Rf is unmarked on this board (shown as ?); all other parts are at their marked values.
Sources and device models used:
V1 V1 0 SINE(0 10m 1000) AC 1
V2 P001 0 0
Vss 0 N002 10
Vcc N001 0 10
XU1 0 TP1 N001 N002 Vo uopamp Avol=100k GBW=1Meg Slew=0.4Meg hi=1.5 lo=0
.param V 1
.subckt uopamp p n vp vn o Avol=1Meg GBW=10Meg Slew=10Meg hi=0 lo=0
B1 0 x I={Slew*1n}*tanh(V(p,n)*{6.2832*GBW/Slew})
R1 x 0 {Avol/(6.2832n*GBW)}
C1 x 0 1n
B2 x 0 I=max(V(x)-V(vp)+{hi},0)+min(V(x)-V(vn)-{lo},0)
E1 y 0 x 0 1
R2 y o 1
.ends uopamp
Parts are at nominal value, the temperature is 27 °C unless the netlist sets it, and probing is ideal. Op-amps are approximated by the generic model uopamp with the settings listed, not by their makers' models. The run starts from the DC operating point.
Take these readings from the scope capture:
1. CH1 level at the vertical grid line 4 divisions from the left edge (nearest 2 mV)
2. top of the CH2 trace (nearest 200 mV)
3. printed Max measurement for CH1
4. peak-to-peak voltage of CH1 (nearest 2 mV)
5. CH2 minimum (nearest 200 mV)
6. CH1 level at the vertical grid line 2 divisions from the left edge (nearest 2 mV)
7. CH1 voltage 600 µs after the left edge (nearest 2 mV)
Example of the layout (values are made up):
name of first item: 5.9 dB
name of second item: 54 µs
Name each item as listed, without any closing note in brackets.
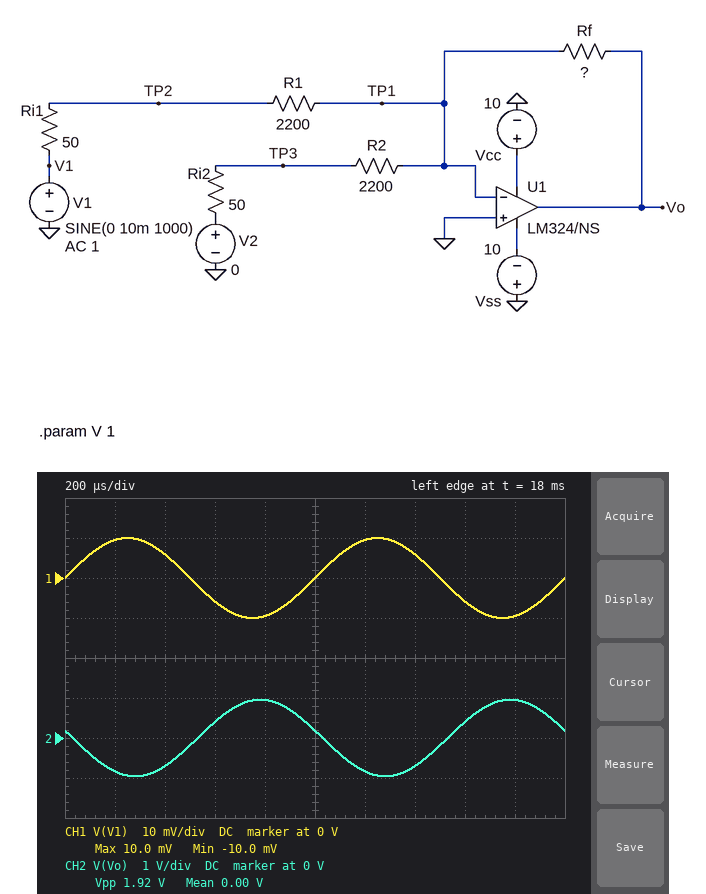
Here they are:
CH1 level at the vertical grid line 4 divisions from the left edge: -10 mV
top of the CH2 trace: 1.0 V
printed Max measurement for CH1: 10.0 mV
peak-to-peak voltage of CH1: 20 mV
CH2 minimum: -1.0 V
CH1 level at the vertical grid line 2 divisions from the left edge: 6 mV
CH1 voltage 600 µs after the left edge: -6 mV
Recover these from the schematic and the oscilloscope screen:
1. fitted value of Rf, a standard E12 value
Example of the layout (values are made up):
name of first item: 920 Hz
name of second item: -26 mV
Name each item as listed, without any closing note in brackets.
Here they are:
fitted value of Rf, a standard E12 value: 220 kΩ
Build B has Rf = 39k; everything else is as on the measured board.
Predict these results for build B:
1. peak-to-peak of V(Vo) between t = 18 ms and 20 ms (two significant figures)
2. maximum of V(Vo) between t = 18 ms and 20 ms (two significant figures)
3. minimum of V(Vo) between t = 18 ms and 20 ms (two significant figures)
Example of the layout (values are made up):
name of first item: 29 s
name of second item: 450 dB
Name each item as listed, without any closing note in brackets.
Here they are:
peak-to-peak of V(Vo) between t = 18 ms and 20 ms: 350 mV
maximum of V(Vo) between t = 18 ms and 20 ms: 170 mV
minimum of V(Vo) between t = 18 ms and 20 ms: -170 mV
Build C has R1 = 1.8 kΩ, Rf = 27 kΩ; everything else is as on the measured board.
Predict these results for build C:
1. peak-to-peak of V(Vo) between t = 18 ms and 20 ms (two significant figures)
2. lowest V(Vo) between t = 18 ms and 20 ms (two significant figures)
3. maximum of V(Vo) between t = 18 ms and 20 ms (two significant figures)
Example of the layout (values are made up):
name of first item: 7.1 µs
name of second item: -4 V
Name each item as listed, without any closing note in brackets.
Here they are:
peak-to-peak of V(Vo) between t = 18 ms and 20 ms: 290 mV
lowest V(Vo) between t = 18 ms and 20 ms: -150 mV
maximum of V(Vo) between t = 18 ms and 20 ms: 150 mV
